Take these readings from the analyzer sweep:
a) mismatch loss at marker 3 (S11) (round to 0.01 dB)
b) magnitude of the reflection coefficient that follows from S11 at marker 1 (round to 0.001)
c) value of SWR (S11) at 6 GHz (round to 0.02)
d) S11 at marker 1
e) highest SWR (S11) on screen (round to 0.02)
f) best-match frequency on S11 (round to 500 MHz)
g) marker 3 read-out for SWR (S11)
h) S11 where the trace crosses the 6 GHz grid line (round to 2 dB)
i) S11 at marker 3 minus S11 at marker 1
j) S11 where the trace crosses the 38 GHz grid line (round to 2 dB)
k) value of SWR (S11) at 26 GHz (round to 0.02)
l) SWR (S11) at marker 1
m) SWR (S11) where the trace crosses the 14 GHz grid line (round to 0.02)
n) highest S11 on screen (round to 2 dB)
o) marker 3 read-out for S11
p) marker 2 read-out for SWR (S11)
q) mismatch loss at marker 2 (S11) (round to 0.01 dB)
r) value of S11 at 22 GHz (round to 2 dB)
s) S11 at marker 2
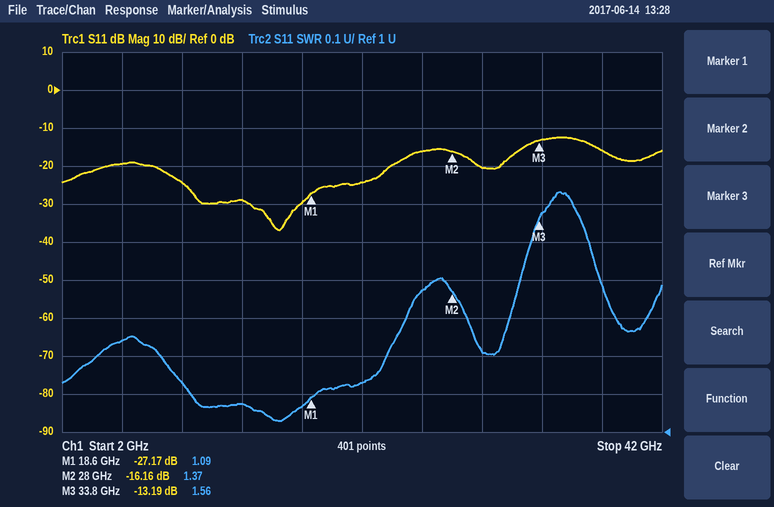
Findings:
0.21 dB
0.044
1.24
-27.17 dB
1.64
16.5 GHz
1.56
-20 dB
13.98 dB
-16 dB
1.38
1.09
1.08
-12 dB
-13.19 dB
1.37
0.11 dB
-24 dB
-16.16 dB
